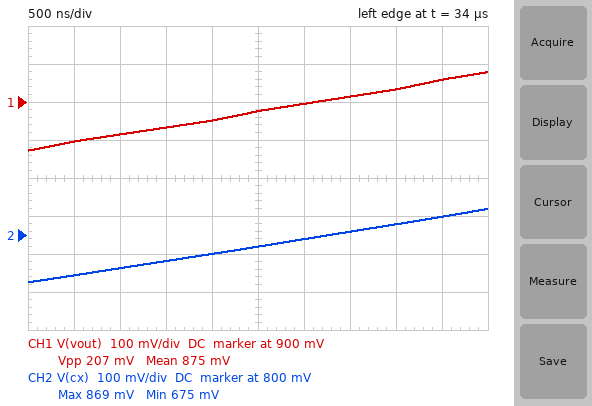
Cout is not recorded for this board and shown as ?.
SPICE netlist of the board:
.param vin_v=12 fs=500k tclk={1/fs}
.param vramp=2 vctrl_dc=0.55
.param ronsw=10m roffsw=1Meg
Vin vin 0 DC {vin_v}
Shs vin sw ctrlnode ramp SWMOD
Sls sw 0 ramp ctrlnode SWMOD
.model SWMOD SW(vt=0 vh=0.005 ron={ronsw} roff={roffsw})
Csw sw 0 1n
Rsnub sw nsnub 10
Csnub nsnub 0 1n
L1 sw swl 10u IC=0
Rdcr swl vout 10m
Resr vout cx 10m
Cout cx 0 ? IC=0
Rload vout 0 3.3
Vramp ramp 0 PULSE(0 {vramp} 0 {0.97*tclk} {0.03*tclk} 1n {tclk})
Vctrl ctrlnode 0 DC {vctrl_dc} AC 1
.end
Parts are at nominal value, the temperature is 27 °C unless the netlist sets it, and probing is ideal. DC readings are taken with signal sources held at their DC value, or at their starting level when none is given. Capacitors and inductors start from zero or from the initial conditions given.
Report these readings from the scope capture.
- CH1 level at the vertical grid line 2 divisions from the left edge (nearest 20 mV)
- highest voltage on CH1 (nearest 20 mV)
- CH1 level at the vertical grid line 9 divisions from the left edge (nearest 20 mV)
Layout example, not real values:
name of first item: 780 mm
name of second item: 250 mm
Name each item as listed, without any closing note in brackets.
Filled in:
CH1 level at the vertical grid line 2 divisions from the left edge: 820 mV
highest voltage on CH1: 980 mV
CH1 level at the vertical grid line 9 divisions from the left edge: 960 mV
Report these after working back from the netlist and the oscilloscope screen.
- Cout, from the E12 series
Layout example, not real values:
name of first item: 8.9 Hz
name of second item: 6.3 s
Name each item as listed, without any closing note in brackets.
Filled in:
Cout, from the E12 series: 270 µF
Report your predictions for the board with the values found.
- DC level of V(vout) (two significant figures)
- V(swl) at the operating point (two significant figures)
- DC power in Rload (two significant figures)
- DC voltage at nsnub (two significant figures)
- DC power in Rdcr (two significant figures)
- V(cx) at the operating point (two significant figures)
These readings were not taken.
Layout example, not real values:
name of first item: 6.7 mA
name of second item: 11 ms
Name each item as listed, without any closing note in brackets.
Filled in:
DC level of V(vout): 12 V
V(swl) at the operating point: 12 V
DC power in Rload: 43 W
DC voltage at nsnub: 12 V
DC power in Rdcr: 130 mW
V(cx) at the operating point: 12 V
